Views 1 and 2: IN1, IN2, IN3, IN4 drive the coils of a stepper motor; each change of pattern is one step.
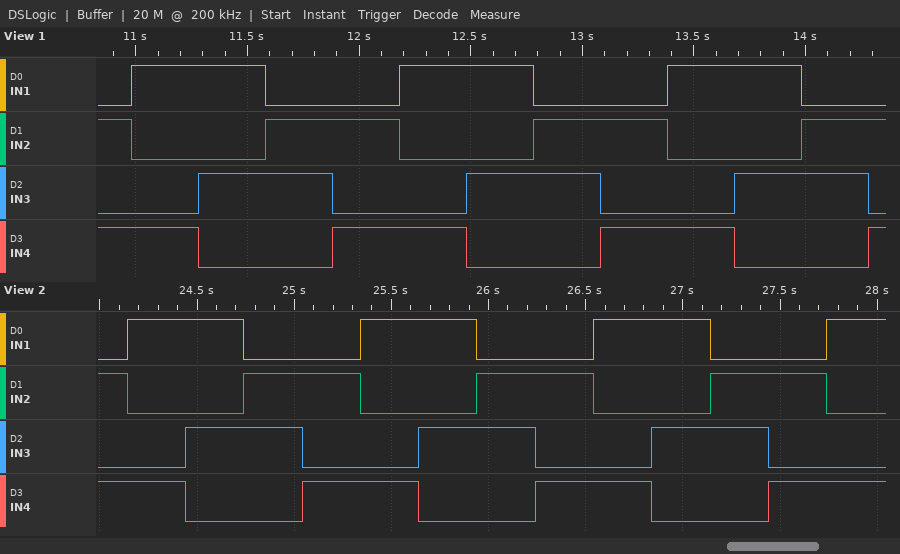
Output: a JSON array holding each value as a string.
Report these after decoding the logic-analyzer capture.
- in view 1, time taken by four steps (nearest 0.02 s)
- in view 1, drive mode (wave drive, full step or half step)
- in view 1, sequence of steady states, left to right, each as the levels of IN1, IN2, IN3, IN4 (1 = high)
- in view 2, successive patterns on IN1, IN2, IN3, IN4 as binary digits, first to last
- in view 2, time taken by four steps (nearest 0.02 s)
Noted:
["1.20 s", "full step", "0101 1001 1010 0110 0101 1001 1010 0110 0101 1001 1010 0110 0101", "0101 1001 1010 0110 0101 1001 1010 0110 0101 1001 1010 0110 0101 1001", "1.20 s"]
